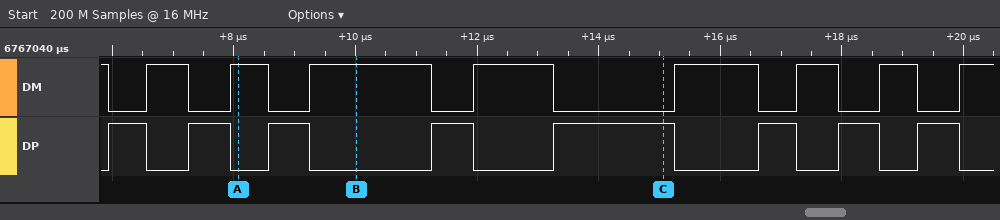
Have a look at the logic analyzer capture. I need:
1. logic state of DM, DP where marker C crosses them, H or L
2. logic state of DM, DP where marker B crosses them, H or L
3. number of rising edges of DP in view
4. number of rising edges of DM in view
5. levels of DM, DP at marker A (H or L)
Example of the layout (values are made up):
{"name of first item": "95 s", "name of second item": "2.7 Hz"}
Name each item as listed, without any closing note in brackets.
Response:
{"logic state of DM, DP where marker C crosses them, H or L": "DM=L, DP=H", "logic state of DM, DP where marker B crosses them, H or L": "DM=H, DP=L", "number of rising edges of DP in view": "8", "number of rising edges of DM in view": "8", "levels of DM, DP at marker A": "DM=H, DP=L"}
